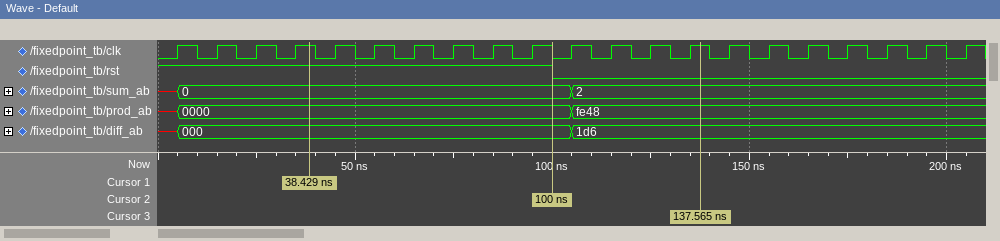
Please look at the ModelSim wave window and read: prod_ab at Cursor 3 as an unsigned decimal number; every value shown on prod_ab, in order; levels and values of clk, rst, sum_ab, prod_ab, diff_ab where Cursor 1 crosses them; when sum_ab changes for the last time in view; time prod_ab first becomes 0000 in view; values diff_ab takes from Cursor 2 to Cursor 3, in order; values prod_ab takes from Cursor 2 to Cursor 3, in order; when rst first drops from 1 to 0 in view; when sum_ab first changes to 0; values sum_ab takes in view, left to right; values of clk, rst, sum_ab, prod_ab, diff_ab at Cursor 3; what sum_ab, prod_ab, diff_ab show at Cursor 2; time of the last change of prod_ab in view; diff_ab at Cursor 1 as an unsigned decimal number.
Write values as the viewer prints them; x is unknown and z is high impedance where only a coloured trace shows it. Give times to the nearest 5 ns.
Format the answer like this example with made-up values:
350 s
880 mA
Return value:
65096
x, 0000, fe48
clk=1, rst=1, sum_ab=0, prod_ab=0000, diff_ab=000
105 ns
5 ns
000, 1d6
0000, fe48
100 ns
5 ns
x, 0, 2
clk=1, rst=0, sum_ab=2, prod_ab=fe48, diff_ab=1d6
sum_ab=0, prod_ab=0000, diff_ab=000
105 ns
0
